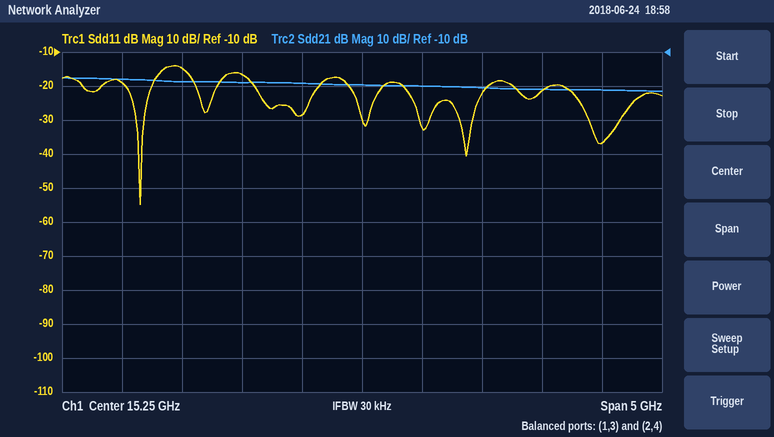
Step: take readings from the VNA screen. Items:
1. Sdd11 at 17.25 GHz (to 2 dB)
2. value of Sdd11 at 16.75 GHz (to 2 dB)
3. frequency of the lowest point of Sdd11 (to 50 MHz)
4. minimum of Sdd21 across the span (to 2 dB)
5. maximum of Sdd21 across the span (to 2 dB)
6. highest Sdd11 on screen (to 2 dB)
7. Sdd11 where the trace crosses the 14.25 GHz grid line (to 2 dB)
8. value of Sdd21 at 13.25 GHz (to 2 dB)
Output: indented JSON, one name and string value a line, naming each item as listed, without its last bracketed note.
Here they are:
{
  "Sdd11 at 17.25 GHz": "-36 dB",
  "value of Sdd11 at 16.75 GHz": "-22 dB",
  "frequency of the lowest point of Sdd11": "13.40 GHz",
  "minimum of Sdd21 across the span": "-22 dB",
  "maximum of Sdd21 across the span": "-18 dB",
  "highest Sdd11 on screen": "-14 dB",
  "Sdd11 where the trace crosses the 14.25 GHz grid line": "-16 dB",
  "value of Sdd21 at 13.25 GHz": "-18 dB"
}
